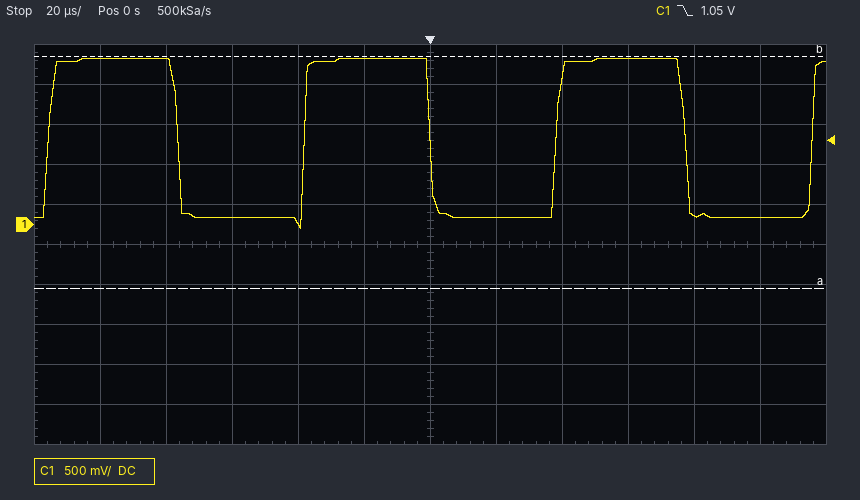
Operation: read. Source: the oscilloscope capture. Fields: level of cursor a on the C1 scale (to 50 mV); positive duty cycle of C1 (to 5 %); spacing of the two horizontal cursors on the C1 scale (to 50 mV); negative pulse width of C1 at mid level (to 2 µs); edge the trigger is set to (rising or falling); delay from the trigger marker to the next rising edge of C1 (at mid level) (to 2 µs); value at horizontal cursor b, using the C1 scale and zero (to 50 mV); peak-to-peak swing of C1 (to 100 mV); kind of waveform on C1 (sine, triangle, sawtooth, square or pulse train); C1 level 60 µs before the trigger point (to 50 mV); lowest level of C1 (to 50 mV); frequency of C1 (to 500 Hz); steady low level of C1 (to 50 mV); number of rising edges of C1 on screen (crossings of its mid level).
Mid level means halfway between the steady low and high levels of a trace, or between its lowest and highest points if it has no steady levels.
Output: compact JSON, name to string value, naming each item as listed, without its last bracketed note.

{"level of cursor a on the C1 scale": "-800 mV", "positive duty cycle of C1": "50 %", "spacing of the two horizontal cursors on the C1 scale": "2.90 V", "negative pulse width of C1 at mid level": "38 µs", "edge the trigger is set to": "falling", "delay from the trigger marker to the next rising edge of C1 (at mid level)": "38 µs", "value at horizontal cursor b, using the C1 scale and zero": "2.10 V", "peak-to-peak swing of C1": "2.10 V", "kind of waveform on C1": "square", "C1 level 60 µs before the trigger point": "100 mV", "lowest level of C1": "-50 mV", "frequency of C1": "13.0 kHz", "steady low level of C1": "100 mV", "number of rising edges of C1 on screen": "4"}
